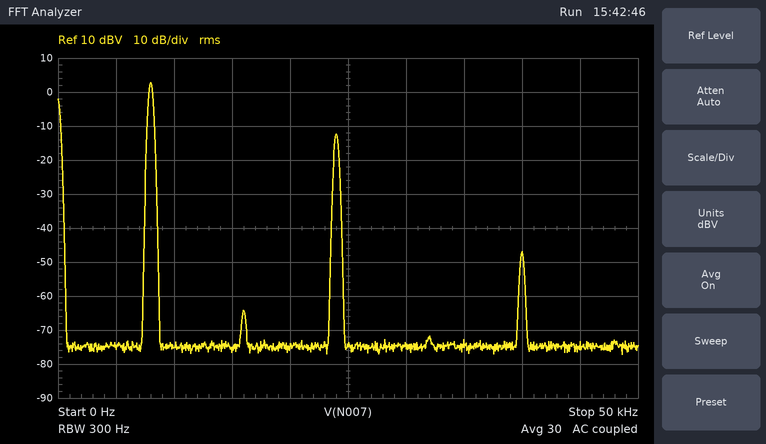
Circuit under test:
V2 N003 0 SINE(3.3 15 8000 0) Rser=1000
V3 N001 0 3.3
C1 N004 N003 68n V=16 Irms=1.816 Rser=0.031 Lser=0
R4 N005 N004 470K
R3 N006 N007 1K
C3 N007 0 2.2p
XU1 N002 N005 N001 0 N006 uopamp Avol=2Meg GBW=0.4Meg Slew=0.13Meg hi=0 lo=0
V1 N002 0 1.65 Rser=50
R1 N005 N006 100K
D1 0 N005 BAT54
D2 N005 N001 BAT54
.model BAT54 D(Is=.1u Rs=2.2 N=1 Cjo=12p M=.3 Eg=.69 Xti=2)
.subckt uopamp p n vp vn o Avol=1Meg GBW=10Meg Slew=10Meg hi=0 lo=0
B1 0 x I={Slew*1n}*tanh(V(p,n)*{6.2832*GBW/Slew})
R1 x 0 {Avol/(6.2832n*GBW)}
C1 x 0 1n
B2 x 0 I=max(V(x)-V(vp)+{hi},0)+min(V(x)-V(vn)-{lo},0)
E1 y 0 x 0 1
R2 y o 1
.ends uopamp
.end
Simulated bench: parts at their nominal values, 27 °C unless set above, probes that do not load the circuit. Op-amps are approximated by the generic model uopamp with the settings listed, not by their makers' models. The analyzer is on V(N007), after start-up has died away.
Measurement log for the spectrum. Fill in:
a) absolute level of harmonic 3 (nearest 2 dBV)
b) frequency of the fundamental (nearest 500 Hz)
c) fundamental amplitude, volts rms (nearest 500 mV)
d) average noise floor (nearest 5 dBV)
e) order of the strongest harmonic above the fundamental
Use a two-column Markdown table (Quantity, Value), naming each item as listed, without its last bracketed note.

| Quantity | Value |
|---|---|
| absolute level of harmonic 3 | -12 dBV |
| frequency of the fundamental | 8.0 kHz |
| fundamental amplitude, volts rms | 1.5 V |
| average noise floor | -75 dBV |
| order of the strongest harmonic above the fundamental | 3 |
